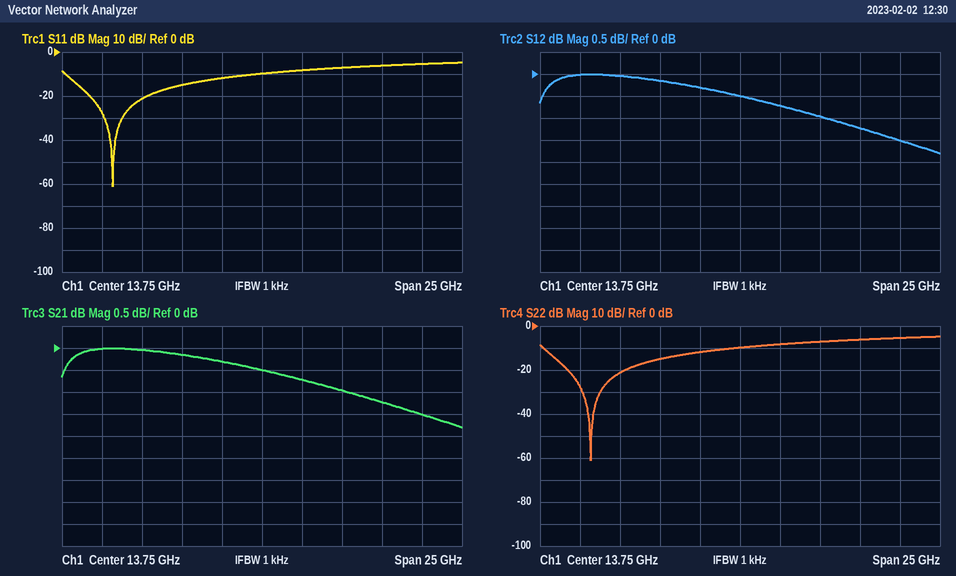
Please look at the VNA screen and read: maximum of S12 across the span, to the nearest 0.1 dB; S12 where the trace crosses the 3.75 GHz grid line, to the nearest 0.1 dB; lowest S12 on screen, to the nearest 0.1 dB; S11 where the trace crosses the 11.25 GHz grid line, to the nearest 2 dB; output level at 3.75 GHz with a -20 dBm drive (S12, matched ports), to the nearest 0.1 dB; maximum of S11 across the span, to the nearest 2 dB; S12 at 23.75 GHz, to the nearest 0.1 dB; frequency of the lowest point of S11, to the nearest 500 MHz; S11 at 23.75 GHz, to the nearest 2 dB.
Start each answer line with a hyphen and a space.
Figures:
- 0.0 dB
- 0.0 dB
- -1.8 dB
- -12 dB
- -20.0 dBm
- -4 dB
- -1.5 dB
- 4.5 GHz
- -6 dB
